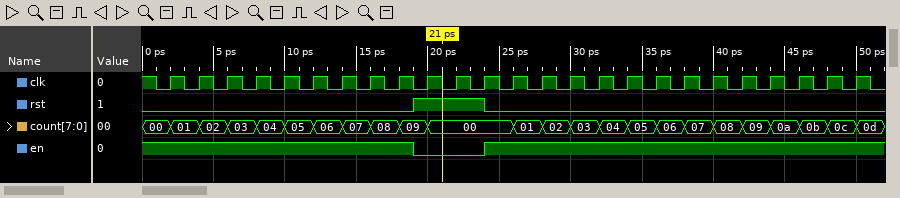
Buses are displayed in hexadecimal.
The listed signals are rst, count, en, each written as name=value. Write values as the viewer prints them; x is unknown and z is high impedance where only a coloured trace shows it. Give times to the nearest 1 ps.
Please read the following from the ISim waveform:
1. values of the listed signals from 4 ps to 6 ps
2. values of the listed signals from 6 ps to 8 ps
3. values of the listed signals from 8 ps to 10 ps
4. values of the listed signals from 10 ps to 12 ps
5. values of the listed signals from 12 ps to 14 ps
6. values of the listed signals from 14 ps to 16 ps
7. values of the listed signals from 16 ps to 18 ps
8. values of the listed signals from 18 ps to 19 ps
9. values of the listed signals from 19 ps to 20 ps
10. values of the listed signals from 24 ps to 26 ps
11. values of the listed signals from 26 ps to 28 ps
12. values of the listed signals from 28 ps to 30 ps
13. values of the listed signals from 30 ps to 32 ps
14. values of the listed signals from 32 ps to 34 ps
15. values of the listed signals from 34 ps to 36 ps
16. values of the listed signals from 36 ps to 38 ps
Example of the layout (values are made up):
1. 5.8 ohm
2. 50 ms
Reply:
1. rst=0, count=02, en=1
2. rst=0, count=03, en=1
3. rst=0, count=04, en=1
4. rst=0, count=05, en=1
5. rst=0, count=06, en=1
6. rst=0, count=07, en=1
7. rst=0, count=08, en=1
8. rst=0, count=09, en=1
9. rst=1, count=09, en=0
10. rst=0, count=00, en=1
11. rst=0, count=01, en=1
12. rst=0, count=02, en=1
13. rst=0, count=03, en=1
14. rst=0, count=04, en=1
15. rst=0, count=05, en=1
16. rst=0, count=06, en=1
